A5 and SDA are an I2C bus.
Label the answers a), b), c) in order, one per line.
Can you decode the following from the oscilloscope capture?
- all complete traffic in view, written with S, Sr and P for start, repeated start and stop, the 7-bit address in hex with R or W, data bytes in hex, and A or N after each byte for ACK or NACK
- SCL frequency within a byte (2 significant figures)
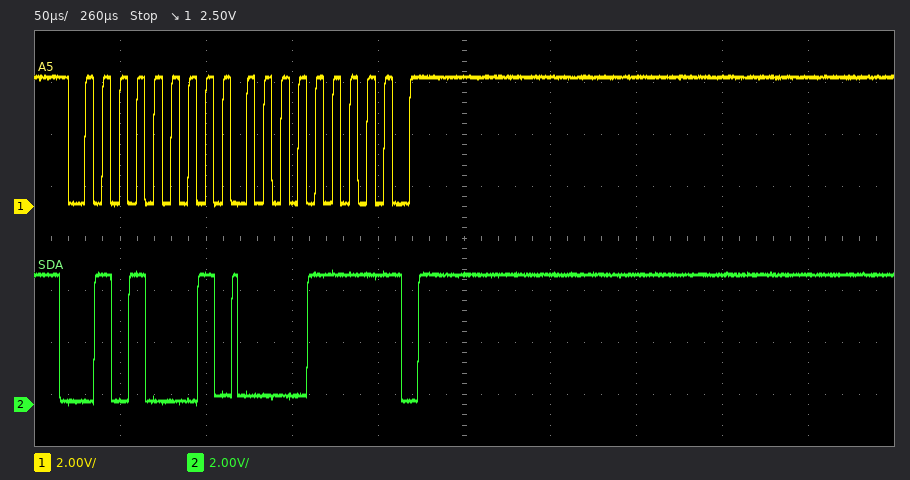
a) S 28R A 0F N P
b) 100 kHz
